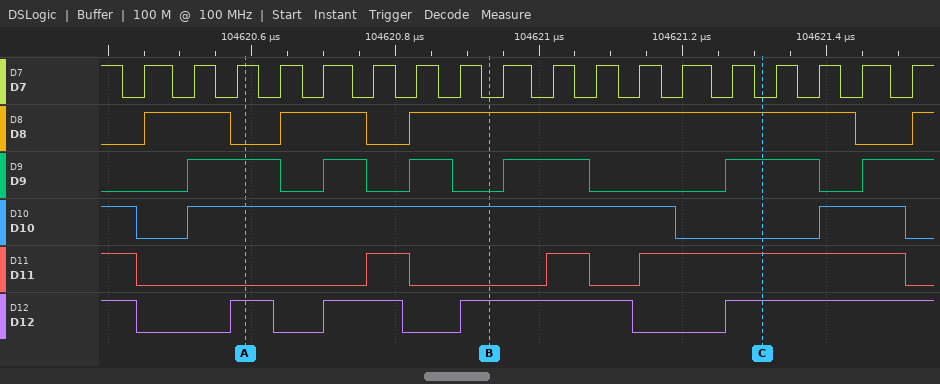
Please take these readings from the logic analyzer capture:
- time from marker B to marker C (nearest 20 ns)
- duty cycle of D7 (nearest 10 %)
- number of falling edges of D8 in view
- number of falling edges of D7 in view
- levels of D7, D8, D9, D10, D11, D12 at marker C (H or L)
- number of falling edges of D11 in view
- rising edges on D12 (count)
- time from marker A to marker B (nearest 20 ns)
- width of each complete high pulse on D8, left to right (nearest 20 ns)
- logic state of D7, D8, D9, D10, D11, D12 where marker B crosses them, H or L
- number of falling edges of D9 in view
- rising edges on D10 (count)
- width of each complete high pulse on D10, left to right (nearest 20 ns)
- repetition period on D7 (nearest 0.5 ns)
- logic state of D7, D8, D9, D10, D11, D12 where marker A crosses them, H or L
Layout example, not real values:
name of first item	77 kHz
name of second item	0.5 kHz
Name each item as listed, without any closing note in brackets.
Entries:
time from marker B to marker C	380 ns
duty cycle of D7	50 %
number of falling edges of D8 in view	3
number of falling edges of D7 in view	18
levels of D7, D8, D9, D10, D11, D12 at marker C	D7=L, D8=H, D9=H, D10=L, D11=H, D12=H
number of falling edges of D11 in view	4
rising edges on D12	4
time from marker A to marker B	340 ns
width of each complete high pulse on D8, left to right	120 ns, 120 ns, 620 ns
logic state of D7, D8, D9, D10, D11, D12 where marker B crosses them, H or L	D7=L, D8=H, D9=L, D10=H, D11=L, D12=H
number of falling edges of D9 in view	5
rising edges on D10	2
width of each complete high pulse on D10, left to right	680 ns, 120 ns
repetition period on D7	63 ns
logic state of D7, D8, D9, D10, D11, D12 where marker A crosses them, H or L	D7=H, D8=L, D9=H, D10=H, D11=L, D12=H
